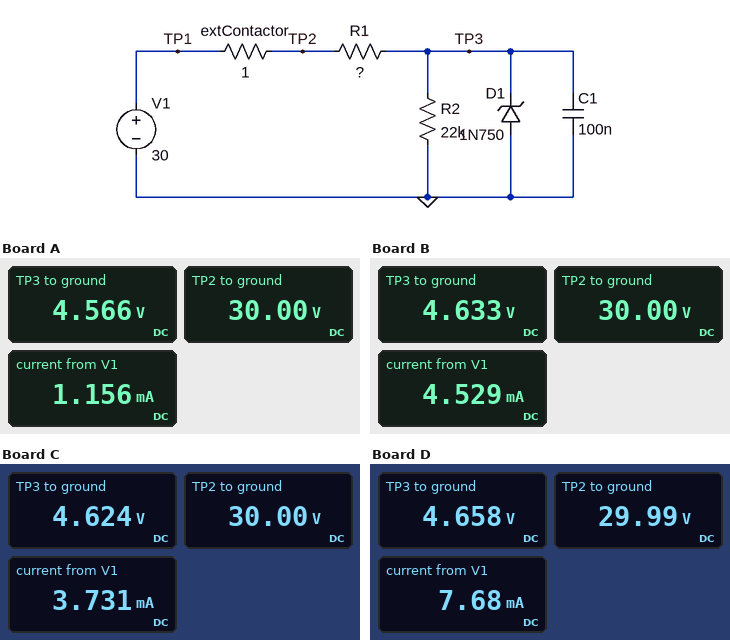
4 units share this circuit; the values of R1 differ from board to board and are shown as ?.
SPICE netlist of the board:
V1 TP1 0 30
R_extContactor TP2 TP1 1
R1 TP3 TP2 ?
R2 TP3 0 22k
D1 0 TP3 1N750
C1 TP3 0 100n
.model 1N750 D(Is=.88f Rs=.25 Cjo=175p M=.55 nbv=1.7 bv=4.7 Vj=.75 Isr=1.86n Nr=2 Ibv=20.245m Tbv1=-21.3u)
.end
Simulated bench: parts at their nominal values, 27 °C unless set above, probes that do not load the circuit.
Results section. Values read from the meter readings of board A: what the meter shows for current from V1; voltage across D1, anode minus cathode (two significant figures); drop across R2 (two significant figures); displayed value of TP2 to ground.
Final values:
1.156 mA
-4.6 V
4.6 V
30.00 V
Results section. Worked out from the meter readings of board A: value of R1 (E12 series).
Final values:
22 kΩ
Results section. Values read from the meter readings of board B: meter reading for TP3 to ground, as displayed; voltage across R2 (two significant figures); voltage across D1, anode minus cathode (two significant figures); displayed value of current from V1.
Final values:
4.633 V
4.6 V
-4.6 V
4.529 mA
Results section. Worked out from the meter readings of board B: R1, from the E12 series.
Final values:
5.6 kΩ
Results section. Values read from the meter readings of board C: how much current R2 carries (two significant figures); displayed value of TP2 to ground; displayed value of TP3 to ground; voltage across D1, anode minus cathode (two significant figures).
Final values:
210 µA
30.00 V
4.624 V
-4.6 V
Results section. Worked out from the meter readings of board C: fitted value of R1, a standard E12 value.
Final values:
6.8 kΩ
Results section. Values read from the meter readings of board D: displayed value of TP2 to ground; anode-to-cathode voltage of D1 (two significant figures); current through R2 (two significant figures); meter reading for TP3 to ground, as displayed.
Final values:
29.99 V
-4.7 V
210 µA
4.658 V
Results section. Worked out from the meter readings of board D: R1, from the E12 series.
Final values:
3.3 kΩ
